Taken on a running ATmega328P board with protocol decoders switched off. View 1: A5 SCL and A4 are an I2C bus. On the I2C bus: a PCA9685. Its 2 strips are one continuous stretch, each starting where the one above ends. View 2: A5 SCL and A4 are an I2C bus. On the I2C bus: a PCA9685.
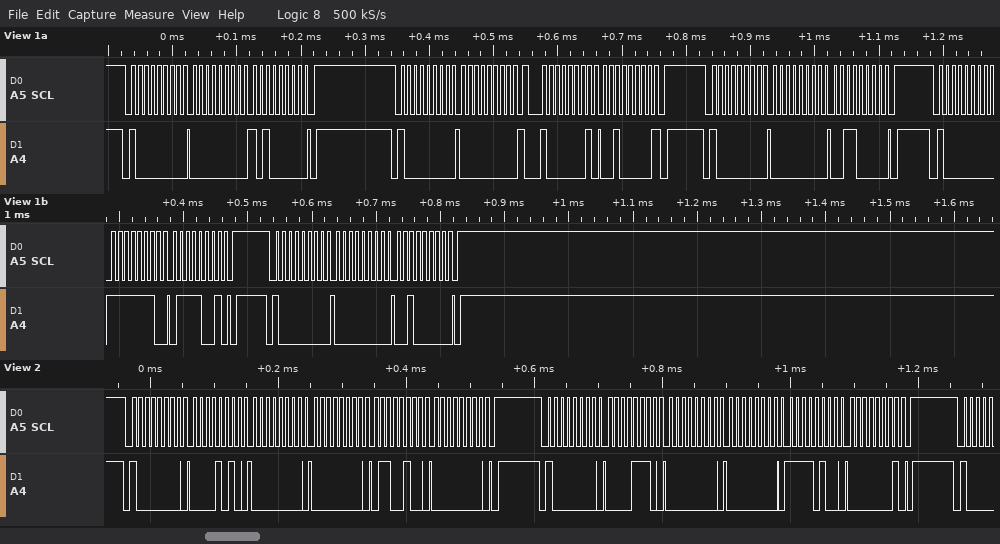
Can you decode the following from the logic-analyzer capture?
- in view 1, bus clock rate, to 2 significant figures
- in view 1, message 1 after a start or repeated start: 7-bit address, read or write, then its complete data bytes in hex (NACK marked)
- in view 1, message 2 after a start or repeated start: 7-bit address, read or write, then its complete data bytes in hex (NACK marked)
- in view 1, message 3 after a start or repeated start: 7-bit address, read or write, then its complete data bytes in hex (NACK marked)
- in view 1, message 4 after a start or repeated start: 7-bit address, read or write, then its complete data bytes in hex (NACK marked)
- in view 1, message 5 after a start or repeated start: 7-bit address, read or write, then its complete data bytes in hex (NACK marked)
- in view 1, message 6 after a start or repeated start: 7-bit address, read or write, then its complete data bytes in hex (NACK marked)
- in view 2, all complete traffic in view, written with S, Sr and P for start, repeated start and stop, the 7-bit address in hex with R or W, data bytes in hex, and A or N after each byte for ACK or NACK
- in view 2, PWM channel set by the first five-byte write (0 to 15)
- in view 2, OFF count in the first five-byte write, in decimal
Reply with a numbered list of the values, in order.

1. 100 kHz
2. 0x40 write: 00 A0
3. 0x40 write: 00
4. 0x40 read: 20 NACK
5. 0x40 write: 00 30
6. 0x40 write: FE 79
7. 0x40 write: 00 20
8. S 40W A 0A A 00 A 00 A 64 A 00 A P S 40W A 0E A 00 A 00 A F4 A 01 A P
9. 1
10. 100
